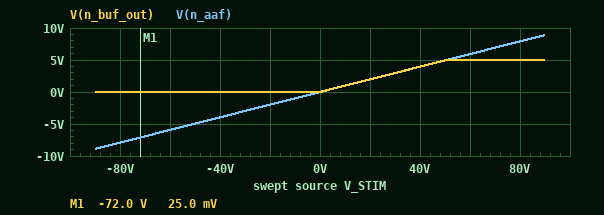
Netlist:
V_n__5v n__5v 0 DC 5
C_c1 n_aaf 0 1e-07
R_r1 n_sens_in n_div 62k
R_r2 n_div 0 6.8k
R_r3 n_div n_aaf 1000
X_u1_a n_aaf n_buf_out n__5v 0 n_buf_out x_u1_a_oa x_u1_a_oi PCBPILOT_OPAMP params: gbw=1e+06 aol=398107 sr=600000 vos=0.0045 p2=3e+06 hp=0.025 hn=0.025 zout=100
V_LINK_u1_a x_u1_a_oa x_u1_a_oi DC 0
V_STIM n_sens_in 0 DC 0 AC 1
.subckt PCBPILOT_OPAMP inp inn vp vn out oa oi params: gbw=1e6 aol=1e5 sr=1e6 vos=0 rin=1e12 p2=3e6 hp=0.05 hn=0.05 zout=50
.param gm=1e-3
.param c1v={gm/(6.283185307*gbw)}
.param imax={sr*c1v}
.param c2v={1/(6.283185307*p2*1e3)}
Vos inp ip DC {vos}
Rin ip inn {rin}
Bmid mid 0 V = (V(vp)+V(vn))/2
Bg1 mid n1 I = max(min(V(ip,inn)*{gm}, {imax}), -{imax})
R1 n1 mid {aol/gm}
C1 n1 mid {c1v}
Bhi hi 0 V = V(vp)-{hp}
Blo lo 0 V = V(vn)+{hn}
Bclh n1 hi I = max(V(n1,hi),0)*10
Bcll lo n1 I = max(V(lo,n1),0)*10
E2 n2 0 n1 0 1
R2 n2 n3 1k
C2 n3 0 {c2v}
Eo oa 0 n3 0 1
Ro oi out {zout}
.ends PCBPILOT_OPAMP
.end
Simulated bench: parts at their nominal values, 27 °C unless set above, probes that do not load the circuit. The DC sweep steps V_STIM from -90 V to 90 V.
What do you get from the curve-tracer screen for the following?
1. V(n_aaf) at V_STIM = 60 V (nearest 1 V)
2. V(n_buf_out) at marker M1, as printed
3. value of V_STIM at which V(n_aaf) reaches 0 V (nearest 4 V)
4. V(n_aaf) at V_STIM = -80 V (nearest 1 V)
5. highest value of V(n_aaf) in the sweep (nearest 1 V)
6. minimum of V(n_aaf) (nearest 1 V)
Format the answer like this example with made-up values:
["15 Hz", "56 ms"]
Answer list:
["6 V", "25.0 mV", "0 V", "-8 V", "9 V", "-9 V"]
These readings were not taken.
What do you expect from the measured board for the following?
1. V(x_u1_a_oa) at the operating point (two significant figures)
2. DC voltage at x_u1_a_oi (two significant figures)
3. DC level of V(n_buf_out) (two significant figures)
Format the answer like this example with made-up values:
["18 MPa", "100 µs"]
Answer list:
["25 mV", "25 mV", "25 mV"]
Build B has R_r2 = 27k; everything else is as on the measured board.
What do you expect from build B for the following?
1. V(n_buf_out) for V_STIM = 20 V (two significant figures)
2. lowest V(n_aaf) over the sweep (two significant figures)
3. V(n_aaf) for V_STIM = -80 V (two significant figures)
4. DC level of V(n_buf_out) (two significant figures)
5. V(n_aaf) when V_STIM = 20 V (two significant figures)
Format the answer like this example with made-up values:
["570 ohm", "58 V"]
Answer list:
["5.0 V", "-27 V", "-24 V", "25 mV", "6.1 V"]
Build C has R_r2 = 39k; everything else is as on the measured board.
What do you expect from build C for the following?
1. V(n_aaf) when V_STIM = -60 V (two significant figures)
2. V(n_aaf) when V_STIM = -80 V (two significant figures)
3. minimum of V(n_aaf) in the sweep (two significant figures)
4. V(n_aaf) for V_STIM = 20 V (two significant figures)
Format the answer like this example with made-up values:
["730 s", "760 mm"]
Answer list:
["-23 V", "-31 V", "-35 V", "7.7 V"]
